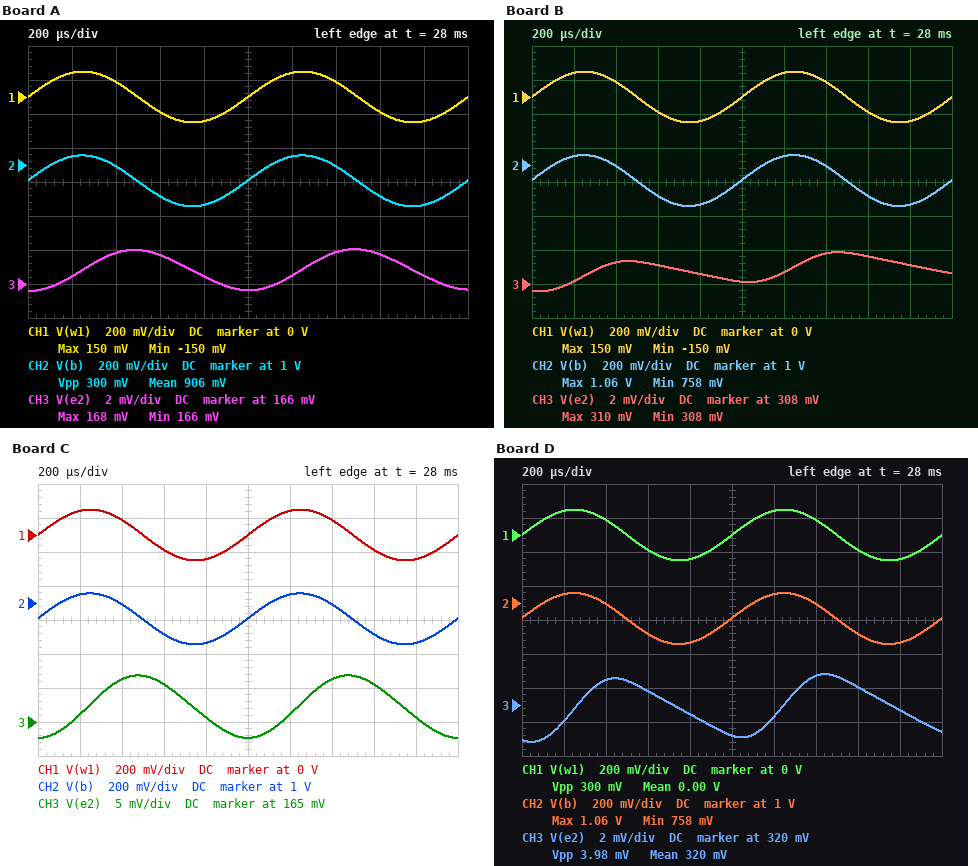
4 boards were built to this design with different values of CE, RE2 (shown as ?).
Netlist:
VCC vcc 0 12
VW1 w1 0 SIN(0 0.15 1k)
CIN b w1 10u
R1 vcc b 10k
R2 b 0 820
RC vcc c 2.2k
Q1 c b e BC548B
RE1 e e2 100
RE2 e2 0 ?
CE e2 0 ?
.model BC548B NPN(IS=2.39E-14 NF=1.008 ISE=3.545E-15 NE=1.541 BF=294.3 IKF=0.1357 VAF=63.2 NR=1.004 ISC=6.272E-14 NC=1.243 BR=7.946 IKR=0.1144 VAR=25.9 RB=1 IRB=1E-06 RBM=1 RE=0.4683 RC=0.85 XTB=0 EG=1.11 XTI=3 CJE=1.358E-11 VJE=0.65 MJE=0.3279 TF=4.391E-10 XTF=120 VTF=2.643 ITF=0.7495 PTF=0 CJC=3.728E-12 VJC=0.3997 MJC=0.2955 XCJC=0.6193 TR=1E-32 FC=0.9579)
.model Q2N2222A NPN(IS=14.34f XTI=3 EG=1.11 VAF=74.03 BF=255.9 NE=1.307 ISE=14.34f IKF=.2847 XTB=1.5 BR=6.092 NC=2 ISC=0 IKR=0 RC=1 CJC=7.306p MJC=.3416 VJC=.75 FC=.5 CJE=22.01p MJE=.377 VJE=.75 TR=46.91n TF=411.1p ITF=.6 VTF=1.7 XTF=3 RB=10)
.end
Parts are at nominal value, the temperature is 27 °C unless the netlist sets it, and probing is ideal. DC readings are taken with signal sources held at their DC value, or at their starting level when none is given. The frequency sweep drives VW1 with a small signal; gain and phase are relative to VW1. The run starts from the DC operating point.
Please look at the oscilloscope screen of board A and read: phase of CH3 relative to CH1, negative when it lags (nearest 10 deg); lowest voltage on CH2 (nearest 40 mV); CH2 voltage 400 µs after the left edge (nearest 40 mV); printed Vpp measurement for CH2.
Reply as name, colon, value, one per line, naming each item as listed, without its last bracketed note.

phase of CH3 relative to CH1, negative when it lags: -90 deg
lowest voltage on CH2: 760 mV
CH2 voltage 400 µs after the left edge: 1.00 V
printed Vpp measurement for CH2: 300 mV
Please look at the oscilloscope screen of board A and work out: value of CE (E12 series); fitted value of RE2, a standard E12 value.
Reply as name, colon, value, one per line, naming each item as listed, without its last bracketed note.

value of CE: 150 µF
fitted value of RE2, a standard E12 value: 150 Ω
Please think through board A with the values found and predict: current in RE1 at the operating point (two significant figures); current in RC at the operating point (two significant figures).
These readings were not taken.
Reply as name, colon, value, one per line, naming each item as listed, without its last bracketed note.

current in RE1 at the operating point: 1.1 mA
current in RC at the operating point: 1.1 mA
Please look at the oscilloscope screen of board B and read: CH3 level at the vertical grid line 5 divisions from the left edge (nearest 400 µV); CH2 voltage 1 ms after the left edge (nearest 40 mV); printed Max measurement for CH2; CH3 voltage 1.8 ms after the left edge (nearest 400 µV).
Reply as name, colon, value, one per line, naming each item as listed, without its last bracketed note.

CH3 level at the vertical grid line 5 divisions from the left edge: 308.0 mV
CH2 voltage 1 ms after the left edge: 920 mV
printed Max measurement for CH2: 1.06 V
CH3 voltage 1.8 ms after the left edge: 309.2 mV
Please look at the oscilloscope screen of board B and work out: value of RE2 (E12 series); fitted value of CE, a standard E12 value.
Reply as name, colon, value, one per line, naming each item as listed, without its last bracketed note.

value of RE2: 1 kΩ
fitted value of CE, a standard E12 value: 120 µF
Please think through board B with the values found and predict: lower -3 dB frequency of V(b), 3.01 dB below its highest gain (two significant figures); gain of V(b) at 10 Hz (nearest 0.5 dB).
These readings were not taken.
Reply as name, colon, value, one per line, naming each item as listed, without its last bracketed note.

lower -3 dB frequency of V(b), 3.01 dB below its highest gain: 21 Hz
gain of V(b) at 10 Hz: -7.5 dB
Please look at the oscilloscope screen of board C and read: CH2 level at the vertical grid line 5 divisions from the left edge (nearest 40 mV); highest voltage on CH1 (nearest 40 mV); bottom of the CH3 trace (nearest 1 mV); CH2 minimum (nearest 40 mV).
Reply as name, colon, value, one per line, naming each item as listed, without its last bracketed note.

CH2 level at the vertical grid line 5 divisions from the left edge: 920 mV
highest voltage on CH1: 160 mV
bottom of the CH3 trace: 163 mV
CH2 minimum: 760 mV
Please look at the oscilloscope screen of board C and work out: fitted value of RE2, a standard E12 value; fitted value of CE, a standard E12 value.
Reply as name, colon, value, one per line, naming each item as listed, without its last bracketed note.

fitted value of RE2, a standard E12 value: 150 Ω
fitted value of CE, a standard E12 value: 39 µF
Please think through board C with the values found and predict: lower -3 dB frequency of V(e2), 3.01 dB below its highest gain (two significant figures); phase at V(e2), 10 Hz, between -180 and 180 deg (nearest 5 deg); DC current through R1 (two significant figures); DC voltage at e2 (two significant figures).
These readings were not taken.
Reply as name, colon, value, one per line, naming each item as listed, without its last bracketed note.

lower -3 dB frequency of V(e2), 3.01 dB below its highest gain: 13 Hz
phase at V(e2), 10 Hz, between -180 and 180 deg: 55 deg
DC current through R1: 1.1 mA
DC voltage at e2: 160 mV
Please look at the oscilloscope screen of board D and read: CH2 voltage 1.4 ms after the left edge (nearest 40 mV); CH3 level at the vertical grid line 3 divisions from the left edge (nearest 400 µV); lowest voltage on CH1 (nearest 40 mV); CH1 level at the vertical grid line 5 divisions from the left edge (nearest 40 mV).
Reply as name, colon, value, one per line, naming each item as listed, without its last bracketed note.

CH2 voltage 1.4 ms after the left edge: 1.00 V
CH3 level at the vertical grid line 3 divisions from the left edge: 320.8 mV
lowest voltage on CH1: -160 mV
CH1 level at the vertical grid line 5 divisions from the left edge: 0 V
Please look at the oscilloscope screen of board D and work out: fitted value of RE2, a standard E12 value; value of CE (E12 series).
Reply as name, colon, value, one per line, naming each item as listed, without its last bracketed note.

fitted value of RE2, a standard E12 value: 1 kΩ
value of CE: 47 µF
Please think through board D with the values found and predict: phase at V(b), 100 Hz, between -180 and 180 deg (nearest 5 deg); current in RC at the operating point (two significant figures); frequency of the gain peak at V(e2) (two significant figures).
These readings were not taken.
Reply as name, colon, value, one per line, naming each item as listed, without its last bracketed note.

phase at V(b), 100 Hz, between -180 and 180 deg: 10 deg
current in RC at the operating point: 280 µA
frequency of the gain peak at V(e2): 21 Hz
